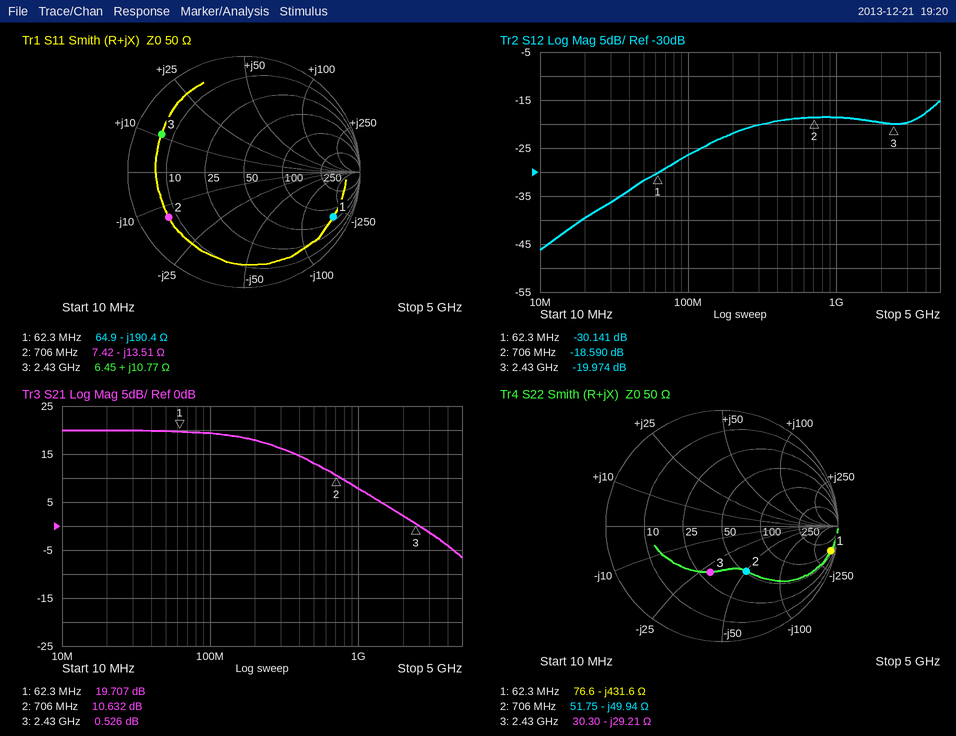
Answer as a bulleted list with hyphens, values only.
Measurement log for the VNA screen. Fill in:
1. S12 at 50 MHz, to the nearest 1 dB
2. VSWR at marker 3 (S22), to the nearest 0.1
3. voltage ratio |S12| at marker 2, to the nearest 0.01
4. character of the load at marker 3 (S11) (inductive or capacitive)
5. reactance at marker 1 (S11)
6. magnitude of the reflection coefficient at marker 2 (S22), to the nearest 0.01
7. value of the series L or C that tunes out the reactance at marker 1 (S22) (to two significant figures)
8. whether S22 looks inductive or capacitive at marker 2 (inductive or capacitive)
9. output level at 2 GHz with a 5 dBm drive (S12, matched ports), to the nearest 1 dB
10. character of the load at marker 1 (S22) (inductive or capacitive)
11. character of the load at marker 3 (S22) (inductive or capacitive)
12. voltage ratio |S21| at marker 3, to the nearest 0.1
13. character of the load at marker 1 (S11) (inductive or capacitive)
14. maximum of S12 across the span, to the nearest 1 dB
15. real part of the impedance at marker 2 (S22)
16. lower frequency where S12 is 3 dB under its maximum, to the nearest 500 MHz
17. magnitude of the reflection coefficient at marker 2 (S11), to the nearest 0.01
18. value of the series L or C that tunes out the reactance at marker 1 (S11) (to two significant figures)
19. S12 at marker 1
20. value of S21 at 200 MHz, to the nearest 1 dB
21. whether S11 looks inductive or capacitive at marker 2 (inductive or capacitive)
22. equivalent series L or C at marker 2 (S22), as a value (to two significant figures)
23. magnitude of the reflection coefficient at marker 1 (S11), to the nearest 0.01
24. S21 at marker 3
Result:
- -32 dB
- 2.4
- 0.12
- inductive
- -190.4 Ω
- 0.44
- 1.1 µH
- capacitive
- -15 dBm
- capacitive
- capacitive
- 1.1
- capacitive
- -15 dB
- 51.75 Ω
- 4.0 GHz
- 0.76
- 490 nH
- -30.141 dB
- 18 dB
- capacitive
- 4.5 pF
- 0.86
- 0.526 dB
